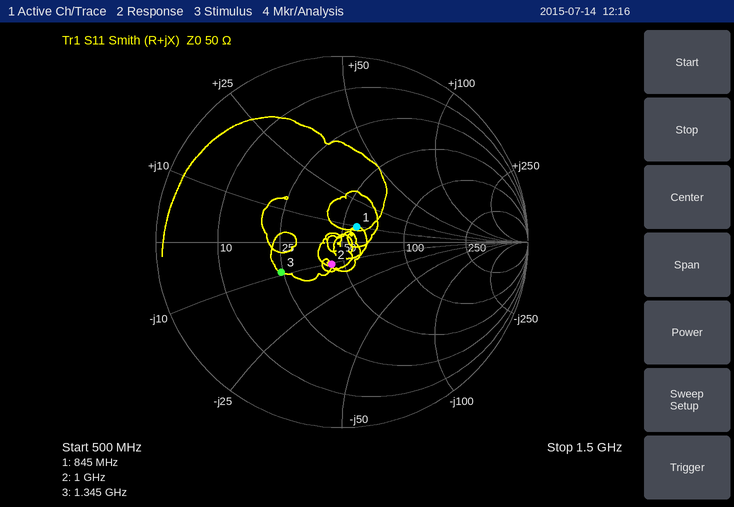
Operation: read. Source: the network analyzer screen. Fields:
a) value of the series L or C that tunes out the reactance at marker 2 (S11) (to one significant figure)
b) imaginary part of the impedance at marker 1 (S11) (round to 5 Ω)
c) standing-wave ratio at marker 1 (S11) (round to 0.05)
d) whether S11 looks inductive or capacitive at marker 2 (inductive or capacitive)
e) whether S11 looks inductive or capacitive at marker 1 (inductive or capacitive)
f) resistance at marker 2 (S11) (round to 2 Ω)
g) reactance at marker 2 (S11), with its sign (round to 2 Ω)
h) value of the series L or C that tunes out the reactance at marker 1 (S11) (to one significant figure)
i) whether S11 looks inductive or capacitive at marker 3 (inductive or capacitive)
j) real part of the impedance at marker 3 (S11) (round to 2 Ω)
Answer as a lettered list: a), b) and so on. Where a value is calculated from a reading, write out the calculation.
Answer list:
a) L = 10 Ω/(2π × 1 GHz) ≈ 2 nH
b) +10 Ω
c) 1.25
d) capacitive
e) inductive
f) 44 Ω
g) -10 Ω
h) C = 1/(2π × 845 MHz × 10 Ω) ≈ 18.8 pF, so 20 pF to one significant figure
i) capacitive
j) 24 Ω
